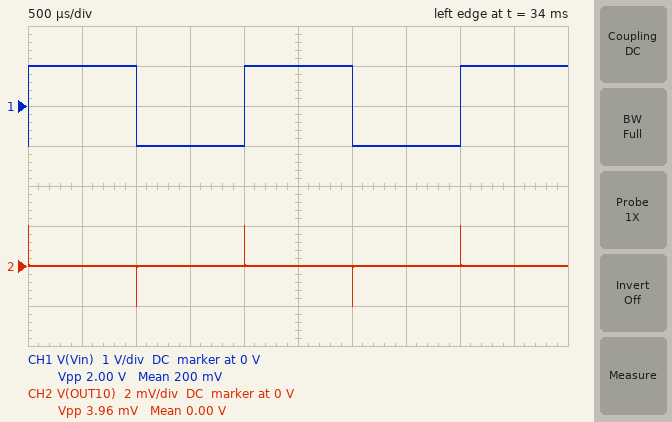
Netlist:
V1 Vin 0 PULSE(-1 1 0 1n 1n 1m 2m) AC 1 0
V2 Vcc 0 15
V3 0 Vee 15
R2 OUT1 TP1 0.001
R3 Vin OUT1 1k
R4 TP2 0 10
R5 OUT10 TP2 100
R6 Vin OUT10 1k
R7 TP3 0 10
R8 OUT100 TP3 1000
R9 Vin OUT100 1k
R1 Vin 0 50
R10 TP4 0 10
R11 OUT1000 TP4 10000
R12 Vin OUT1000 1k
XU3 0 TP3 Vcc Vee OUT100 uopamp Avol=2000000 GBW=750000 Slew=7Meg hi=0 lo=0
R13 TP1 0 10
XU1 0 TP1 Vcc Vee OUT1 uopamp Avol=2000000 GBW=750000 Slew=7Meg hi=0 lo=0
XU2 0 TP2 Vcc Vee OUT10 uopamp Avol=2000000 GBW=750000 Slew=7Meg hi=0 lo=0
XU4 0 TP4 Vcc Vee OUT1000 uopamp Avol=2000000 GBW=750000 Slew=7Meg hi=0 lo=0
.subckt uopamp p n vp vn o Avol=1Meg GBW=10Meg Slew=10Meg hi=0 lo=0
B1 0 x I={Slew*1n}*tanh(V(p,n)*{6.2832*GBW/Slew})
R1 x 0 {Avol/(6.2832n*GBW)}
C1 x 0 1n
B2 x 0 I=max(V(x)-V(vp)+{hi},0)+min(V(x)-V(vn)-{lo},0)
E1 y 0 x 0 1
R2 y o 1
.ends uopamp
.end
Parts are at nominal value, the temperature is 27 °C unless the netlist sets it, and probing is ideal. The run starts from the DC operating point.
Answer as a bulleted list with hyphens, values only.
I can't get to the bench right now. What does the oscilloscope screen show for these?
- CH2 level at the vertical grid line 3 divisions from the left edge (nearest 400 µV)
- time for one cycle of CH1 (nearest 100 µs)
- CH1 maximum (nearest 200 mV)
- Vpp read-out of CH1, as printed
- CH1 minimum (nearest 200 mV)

- 0 V
- 2.0 ms
- 1.0 V
- 2.00 V
- -1.0 V
